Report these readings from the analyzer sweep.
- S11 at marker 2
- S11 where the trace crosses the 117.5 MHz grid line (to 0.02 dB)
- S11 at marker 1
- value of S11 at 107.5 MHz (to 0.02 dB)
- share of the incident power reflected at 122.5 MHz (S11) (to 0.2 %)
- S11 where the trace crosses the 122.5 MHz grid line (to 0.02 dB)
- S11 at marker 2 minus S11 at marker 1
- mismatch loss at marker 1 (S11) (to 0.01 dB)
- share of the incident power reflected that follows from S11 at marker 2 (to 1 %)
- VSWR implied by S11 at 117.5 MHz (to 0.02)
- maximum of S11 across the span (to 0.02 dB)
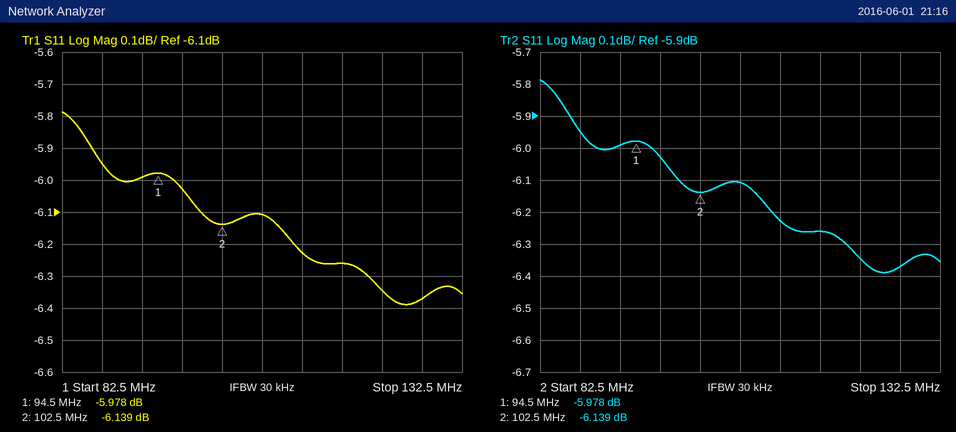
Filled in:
-6.139 dB
-6.26 dB
-5.978 dB
-6.10 dB
23.2 %
-6.34 dB
-0.161 dB
1.26 dB
24 %
2.90
-5.78 dB
